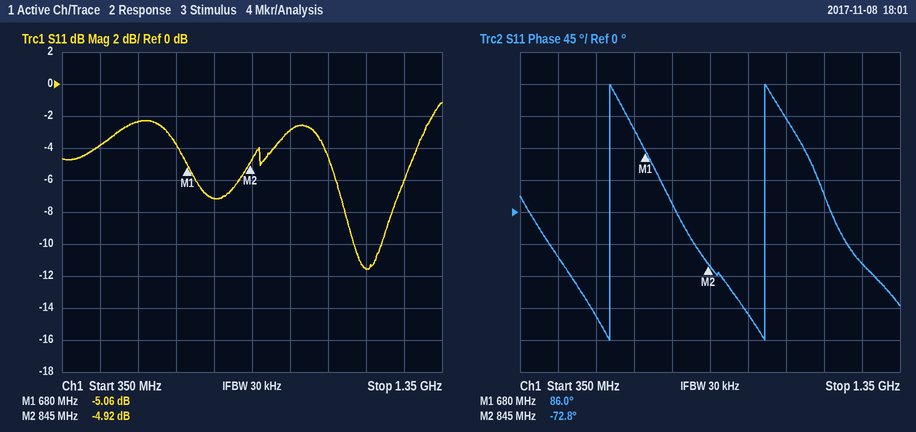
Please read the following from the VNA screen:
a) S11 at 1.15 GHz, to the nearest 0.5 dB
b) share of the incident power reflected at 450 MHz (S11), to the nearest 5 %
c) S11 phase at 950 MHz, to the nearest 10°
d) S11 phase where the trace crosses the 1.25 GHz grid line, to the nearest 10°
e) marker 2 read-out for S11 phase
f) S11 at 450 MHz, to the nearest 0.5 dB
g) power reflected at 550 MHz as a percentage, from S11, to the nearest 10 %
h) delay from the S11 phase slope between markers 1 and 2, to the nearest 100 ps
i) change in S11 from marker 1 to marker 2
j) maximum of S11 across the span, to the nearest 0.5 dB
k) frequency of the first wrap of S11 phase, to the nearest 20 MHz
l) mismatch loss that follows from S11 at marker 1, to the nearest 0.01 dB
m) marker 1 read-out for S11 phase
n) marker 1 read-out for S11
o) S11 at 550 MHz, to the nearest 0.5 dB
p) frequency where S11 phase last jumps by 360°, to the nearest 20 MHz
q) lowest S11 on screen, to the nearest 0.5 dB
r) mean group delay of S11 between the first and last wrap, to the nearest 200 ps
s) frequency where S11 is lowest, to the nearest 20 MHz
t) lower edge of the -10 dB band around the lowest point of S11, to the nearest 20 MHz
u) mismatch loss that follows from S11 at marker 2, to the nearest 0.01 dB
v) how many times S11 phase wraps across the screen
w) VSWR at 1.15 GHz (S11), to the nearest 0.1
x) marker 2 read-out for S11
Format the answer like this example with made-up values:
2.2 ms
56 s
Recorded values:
-11.5 dB
40 %
-140°
-70°
-72.8°
-4.0 dB
60 %
2.7 ns
0.14 dB
-1.0 dB
580 MHz
1.62 dB
86.0°
-5.06 dB
-2.5 dB
1.00 GHz
-11.5 dB
2.4 ns
1.16 GHz
1.12 GHz
1.69 dB
2
1.7
-4.92 dB
